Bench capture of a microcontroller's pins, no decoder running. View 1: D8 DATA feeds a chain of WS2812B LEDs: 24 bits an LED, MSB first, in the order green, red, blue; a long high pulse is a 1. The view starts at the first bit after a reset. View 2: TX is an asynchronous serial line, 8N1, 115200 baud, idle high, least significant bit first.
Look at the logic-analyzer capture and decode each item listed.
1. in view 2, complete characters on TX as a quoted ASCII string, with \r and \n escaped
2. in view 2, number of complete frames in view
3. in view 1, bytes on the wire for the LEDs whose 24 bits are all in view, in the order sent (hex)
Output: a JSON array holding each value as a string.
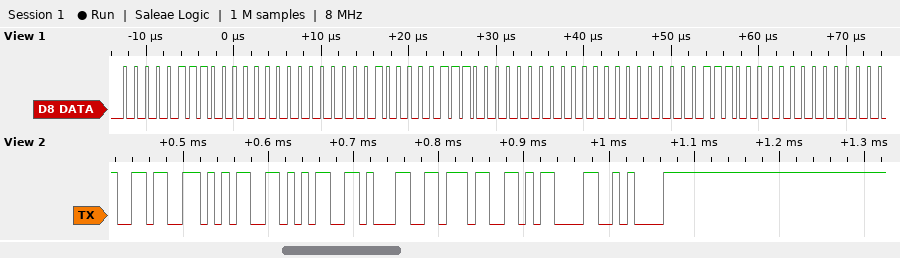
["\"65517\\r\\n\"", "7", "07 00 01 07 00 00"]
